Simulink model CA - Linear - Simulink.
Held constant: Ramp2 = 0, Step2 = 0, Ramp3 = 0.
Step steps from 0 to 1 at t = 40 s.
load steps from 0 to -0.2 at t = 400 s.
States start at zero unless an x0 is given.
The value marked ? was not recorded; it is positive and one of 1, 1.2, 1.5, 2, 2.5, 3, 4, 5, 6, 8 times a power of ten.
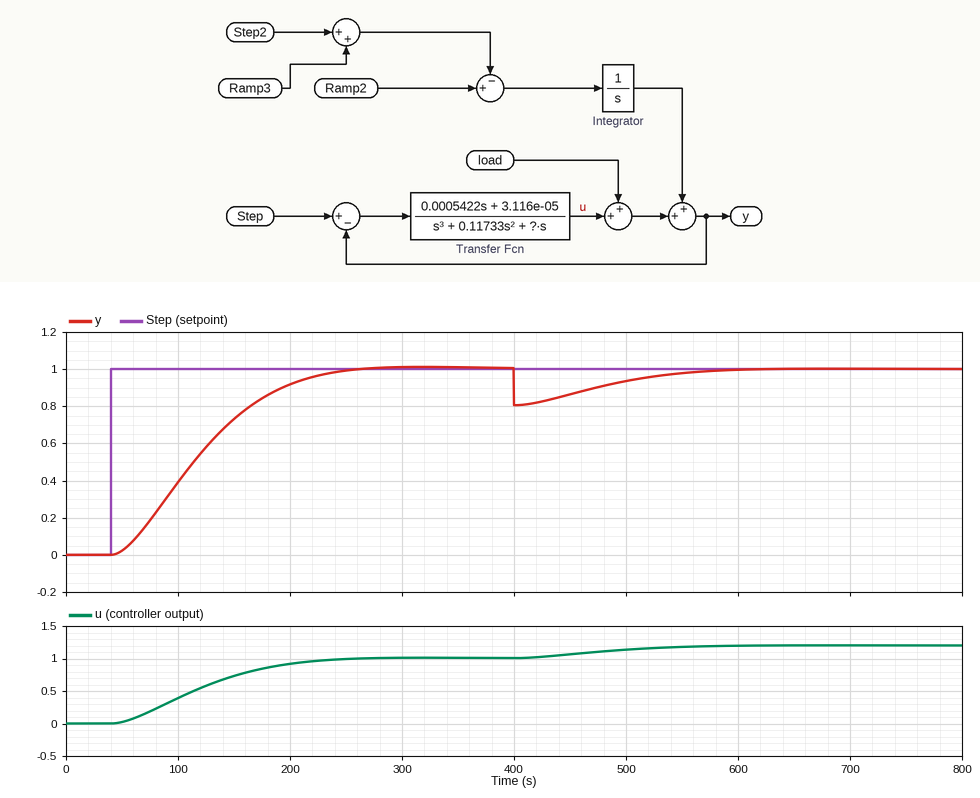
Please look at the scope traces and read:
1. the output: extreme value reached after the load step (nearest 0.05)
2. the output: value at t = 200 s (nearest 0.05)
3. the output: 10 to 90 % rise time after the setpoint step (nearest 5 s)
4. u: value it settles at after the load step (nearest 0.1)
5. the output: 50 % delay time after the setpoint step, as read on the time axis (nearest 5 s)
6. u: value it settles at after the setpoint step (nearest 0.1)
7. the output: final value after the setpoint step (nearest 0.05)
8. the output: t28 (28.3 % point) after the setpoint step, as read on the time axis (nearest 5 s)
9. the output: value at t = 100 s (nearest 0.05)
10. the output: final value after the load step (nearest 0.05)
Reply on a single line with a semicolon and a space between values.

0.80; 0.90; 130 s; 1.2; 115 s; 1.0; 1.00; 85 s; 0.40; 1.00
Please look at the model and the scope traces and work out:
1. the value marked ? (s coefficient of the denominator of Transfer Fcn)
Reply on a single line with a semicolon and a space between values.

0.0025
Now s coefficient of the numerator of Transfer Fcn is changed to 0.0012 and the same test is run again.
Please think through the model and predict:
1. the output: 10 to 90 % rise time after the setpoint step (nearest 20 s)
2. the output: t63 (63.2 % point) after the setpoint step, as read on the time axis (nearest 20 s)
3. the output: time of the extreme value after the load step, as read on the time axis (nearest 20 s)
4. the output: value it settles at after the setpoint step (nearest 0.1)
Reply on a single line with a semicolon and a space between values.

160 s; 120 s; 400 s; 1.0
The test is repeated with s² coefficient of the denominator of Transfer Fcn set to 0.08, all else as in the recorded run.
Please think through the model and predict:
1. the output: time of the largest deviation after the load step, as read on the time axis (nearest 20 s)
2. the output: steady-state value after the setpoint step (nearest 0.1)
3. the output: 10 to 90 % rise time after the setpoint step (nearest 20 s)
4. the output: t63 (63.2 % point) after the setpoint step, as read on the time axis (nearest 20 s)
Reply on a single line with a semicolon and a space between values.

400 s; 1.0; 140 s; 120 s
